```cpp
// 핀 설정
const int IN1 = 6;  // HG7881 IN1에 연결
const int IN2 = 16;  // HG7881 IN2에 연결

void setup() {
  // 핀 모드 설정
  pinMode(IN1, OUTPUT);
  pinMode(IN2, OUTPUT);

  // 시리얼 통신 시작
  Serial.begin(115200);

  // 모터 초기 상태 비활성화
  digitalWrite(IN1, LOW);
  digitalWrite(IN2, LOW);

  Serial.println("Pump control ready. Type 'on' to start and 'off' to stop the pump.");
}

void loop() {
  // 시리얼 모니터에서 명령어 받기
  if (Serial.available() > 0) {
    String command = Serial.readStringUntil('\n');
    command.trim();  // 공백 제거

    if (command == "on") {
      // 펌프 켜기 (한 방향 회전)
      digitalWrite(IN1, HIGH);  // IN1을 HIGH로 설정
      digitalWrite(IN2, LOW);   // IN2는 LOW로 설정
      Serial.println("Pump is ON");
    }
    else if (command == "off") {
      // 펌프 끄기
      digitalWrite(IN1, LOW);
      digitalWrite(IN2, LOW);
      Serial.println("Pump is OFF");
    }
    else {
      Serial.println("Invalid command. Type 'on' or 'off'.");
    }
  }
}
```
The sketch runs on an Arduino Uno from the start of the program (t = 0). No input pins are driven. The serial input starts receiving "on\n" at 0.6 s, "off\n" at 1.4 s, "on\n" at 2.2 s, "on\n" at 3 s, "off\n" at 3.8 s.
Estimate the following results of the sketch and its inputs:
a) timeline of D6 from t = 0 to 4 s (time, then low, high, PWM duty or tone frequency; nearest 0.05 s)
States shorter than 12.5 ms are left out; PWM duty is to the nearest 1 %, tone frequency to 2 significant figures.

0 s low; 0.6 s high; 1.4 s low; 2.2 s high; 3.8 s low
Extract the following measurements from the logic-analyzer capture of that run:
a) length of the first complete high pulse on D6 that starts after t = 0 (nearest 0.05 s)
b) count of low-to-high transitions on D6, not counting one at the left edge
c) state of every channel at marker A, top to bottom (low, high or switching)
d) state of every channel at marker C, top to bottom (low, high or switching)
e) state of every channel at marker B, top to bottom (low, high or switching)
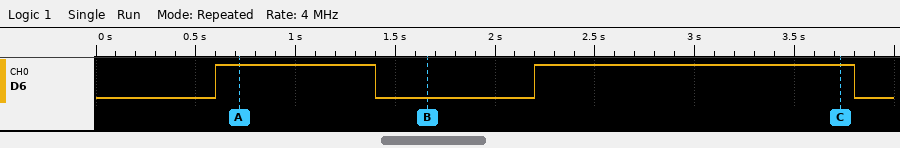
0.80 s
2
D6 high
D6 high
D6 low
